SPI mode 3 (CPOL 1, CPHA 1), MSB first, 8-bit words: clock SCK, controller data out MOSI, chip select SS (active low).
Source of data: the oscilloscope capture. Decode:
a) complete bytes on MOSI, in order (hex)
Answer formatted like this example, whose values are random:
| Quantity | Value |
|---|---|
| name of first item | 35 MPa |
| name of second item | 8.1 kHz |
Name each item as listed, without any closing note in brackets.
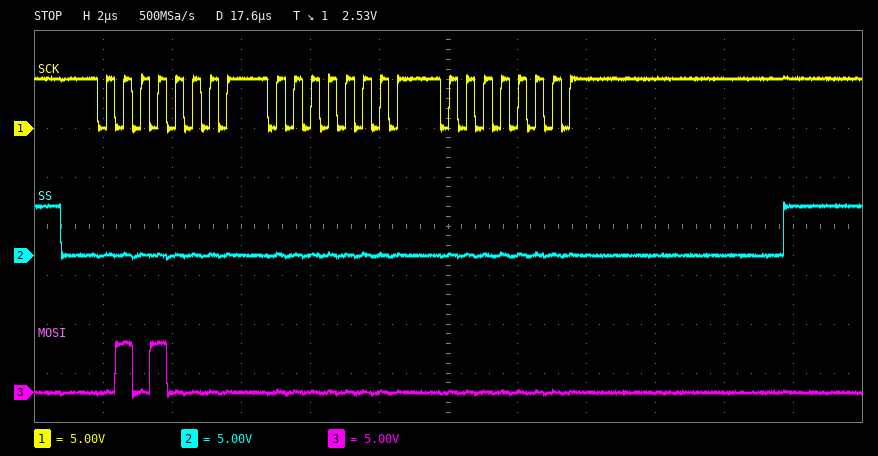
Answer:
| Quantity | Value |
|---|---|
| complete bytes on MOSI, in order | 50 00 00 |
